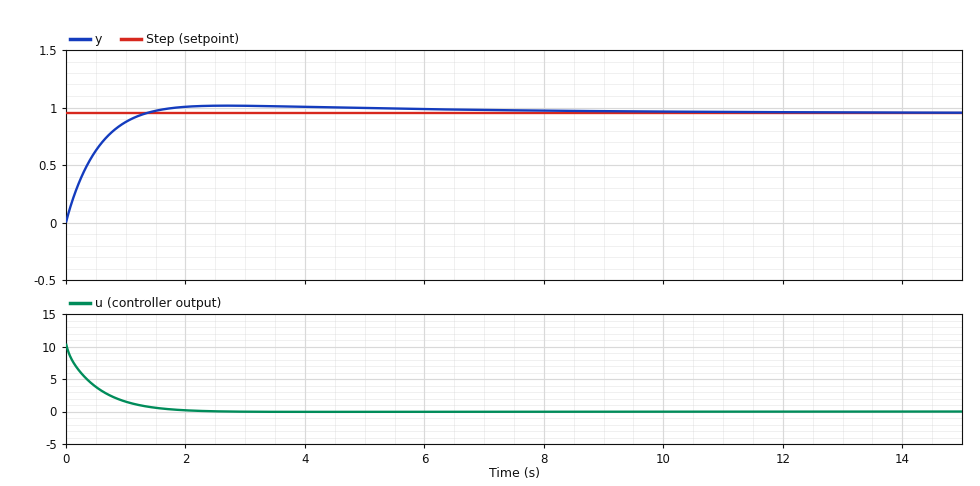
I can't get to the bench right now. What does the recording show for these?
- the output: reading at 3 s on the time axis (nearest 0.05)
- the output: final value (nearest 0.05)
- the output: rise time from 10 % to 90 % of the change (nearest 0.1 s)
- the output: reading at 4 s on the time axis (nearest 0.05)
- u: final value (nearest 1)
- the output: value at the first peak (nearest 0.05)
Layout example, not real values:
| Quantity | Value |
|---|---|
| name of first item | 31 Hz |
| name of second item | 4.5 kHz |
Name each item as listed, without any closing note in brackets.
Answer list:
| Quantity | Value |
|---|---|
| the output: reading at 3 s on the time axis | 1.00 |
| the output: final value | 0.95 |
| the output: rise time from 10 % to 90 % of the change | 0.9 s |
| the output: reading at 4 s on the time axis | 1.00 |
| u: final value | 0 |
| the output: value at the first peak | 1.00 |
